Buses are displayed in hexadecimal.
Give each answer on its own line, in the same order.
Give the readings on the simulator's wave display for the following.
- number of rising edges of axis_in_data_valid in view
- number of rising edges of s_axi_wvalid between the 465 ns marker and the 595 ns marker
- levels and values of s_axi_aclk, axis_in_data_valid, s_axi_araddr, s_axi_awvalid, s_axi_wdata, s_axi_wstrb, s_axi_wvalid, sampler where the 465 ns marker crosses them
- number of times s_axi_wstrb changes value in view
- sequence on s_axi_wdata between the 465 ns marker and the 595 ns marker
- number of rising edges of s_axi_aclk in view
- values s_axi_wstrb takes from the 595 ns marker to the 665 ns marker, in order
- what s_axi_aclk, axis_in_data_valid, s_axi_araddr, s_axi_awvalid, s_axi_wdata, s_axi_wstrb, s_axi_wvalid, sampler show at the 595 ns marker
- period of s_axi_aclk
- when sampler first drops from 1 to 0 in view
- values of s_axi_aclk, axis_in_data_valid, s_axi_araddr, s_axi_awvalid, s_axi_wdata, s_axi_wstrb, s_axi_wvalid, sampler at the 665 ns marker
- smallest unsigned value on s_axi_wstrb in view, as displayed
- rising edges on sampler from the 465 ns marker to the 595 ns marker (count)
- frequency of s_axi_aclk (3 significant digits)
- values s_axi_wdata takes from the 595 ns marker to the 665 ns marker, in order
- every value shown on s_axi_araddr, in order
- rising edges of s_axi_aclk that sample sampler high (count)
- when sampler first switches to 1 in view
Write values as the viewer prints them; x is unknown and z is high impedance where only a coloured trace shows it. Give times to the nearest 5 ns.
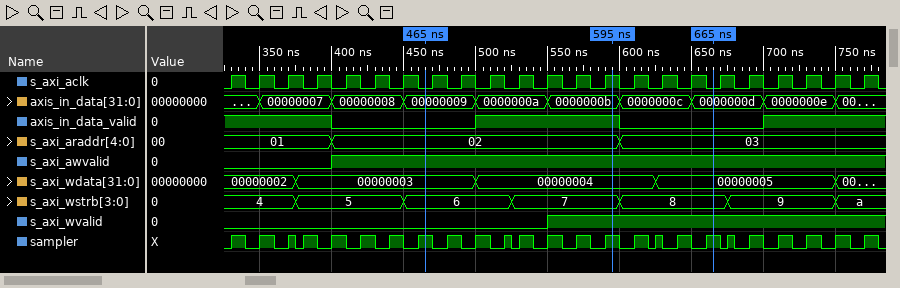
2
1
s_axi_aclk=0, axis_in_data_valid=0, s_axi_araddr=02, s_axi_awvalid=1, s_axi_wdata=00000003, s_axi_wstrb=6, s_axi_wvalid=0, sampler=1
6
00000003, 00000004
23
7, 8
s_axi_aclk=1, axis_in_data_valid=1, s_axi_araddr=02, s_axi_awvalid=1, s_axi_wdata=00000004, s_axi_wstrb=7, s_axi_wvalid=1, sampler=1
20 ns
340 ns
s_axi_aclk=0, axis_in_data_valid=0, s_axi_araddr=03, s_axi_awvalid=1, s_axi_wdata=00000005, s_axi_wstrb=8, s_axi_wvalid=1, sampler=1
4
7
50.0 MHz
00000004, 00000005
01, 02, 03
10
330 ns
